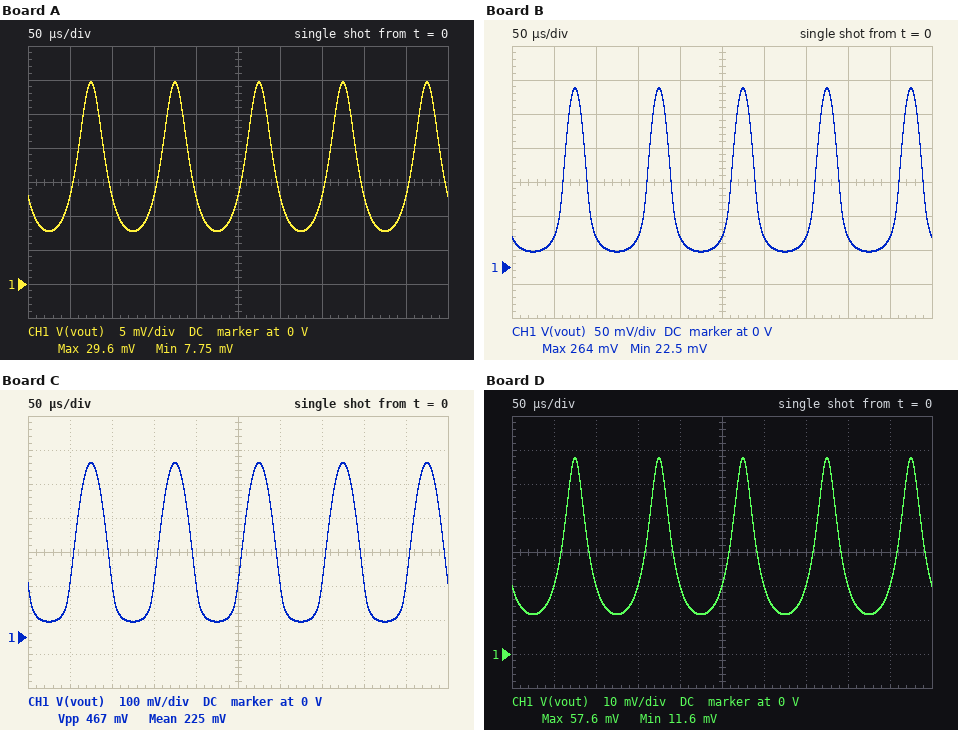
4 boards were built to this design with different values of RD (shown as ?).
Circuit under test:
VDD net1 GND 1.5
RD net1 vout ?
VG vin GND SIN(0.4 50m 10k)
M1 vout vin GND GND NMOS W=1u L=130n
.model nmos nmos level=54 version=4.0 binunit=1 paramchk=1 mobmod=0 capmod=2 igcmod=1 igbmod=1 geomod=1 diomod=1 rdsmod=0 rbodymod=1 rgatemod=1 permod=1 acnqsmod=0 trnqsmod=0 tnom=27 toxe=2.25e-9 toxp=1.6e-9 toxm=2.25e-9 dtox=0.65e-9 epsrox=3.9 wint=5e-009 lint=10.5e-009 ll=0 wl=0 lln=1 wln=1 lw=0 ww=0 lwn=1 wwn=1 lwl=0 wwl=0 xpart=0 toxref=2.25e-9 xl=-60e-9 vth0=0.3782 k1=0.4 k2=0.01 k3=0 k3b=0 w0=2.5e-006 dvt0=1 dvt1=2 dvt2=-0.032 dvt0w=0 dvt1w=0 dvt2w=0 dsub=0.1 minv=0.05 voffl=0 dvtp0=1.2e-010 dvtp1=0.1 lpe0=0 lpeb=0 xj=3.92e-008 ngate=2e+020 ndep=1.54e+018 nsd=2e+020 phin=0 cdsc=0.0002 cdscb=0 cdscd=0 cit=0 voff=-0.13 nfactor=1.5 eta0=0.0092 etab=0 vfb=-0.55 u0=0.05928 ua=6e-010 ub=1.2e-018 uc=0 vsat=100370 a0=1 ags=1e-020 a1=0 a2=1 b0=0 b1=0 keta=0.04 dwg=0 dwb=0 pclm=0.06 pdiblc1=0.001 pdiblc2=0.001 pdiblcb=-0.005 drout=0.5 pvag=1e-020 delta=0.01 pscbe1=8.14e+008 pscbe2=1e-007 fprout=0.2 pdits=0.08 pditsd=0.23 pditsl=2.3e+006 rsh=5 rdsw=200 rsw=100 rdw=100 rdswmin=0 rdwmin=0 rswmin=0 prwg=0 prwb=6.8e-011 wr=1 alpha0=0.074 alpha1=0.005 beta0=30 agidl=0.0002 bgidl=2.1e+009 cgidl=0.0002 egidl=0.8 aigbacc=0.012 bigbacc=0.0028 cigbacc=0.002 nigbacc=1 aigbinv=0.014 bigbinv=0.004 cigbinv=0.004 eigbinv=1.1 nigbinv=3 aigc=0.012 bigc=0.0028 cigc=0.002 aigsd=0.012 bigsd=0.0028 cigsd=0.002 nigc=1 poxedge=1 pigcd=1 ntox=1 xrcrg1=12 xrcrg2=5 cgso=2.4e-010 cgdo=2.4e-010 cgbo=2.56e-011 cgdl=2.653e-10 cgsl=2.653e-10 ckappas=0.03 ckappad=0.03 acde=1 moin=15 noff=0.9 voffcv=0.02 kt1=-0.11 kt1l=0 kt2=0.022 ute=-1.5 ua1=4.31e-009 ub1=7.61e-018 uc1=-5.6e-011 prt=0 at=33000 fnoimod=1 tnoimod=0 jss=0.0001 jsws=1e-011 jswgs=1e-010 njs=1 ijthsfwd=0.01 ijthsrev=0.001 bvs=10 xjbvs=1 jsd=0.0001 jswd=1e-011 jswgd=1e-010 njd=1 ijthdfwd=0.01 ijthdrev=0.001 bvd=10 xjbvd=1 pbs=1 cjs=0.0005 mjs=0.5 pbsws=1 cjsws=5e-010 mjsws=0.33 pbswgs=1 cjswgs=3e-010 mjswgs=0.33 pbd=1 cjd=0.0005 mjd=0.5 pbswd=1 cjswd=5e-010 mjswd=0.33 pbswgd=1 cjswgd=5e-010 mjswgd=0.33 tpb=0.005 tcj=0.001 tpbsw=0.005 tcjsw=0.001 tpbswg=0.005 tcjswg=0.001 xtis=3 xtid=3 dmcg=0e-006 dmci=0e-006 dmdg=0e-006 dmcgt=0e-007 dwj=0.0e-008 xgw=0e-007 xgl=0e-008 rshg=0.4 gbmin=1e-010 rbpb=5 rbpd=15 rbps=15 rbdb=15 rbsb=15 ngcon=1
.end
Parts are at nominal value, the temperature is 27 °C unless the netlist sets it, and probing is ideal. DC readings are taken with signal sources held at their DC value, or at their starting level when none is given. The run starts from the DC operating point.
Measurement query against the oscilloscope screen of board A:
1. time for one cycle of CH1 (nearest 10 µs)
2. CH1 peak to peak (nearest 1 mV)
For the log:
100 µs
22 mV
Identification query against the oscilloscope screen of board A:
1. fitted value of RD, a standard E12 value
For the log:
220 kΩ
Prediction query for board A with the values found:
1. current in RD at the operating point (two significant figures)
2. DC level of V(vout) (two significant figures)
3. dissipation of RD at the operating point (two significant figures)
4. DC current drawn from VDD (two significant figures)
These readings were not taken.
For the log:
6.8 µA
13 mV
10 µW
6.8 µA
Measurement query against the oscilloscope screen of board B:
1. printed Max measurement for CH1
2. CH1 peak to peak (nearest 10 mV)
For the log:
264 mV
240 mV
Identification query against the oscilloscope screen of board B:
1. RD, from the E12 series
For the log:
82 kΩ
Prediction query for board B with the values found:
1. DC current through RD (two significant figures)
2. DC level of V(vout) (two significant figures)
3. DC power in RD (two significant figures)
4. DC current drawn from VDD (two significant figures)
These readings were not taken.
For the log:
18 µA
44 mV
26 µW
18 µA
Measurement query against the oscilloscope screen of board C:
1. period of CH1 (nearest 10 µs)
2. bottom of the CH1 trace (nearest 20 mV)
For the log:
100 µs
40 mV
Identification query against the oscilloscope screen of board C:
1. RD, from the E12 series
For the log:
47 kΩ
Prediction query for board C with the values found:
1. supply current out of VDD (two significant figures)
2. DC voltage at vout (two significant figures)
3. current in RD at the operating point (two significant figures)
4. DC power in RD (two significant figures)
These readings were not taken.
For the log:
29 µA
160 mV
29 µA
38 µW
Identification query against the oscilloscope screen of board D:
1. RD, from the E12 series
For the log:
150 kΩ
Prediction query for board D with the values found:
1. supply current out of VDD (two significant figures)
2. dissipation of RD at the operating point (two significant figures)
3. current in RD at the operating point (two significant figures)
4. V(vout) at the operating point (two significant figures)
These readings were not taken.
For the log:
9.9 µA
15 µW
9.9 µA
20 mV
